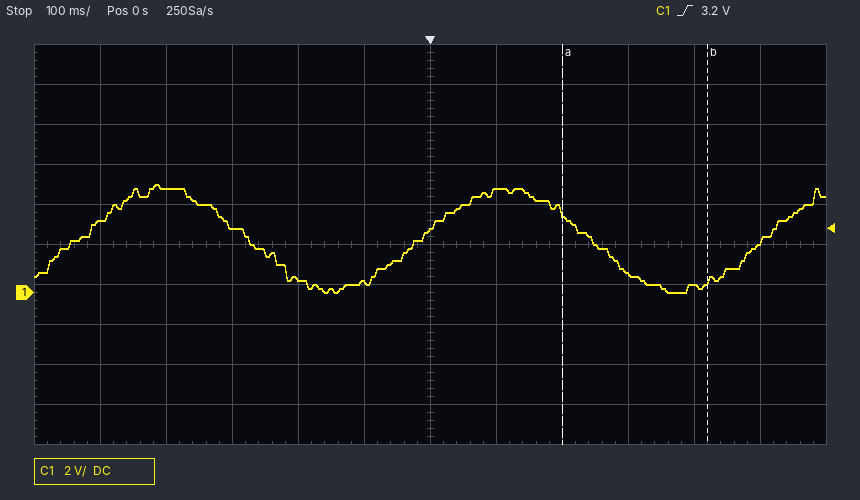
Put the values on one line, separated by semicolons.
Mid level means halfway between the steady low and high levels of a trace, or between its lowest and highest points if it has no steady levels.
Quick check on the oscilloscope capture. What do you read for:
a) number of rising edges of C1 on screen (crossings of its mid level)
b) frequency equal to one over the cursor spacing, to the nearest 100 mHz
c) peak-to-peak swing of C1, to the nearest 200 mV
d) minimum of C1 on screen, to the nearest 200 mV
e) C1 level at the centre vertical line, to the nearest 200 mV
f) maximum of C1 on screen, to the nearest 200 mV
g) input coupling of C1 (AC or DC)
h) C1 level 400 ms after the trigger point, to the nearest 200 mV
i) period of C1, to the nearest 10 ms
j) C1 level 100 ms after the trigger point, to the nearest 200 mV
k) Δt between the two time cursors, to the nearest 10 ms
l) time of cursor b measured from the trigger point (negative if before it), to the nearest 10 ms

3; 4.5 Hz; 5.4 V; 0.0 V; 3.2 V; 5.4 V; DC; 400 mV; 520 ms; 5.2 V; 220 ms; +420 ms
